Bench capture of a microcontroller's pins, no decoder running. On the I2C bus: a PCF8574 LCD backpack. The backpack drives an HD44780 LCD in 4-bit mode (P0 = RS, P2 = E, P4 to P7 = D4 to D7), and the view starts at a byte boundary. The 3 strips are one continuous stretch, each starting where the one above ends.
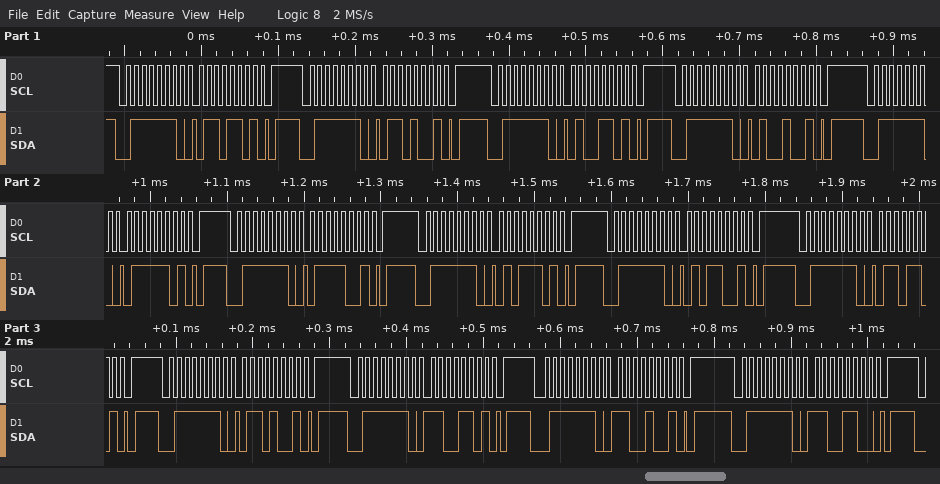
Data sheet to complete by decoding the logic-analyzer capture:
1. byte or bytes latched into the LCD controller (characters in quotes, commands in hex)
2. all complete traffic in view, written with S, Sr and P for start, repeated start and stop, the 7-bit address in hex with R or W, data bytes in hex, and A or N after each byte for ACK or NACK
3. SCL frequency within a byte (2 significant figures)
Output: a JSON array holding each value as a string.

["'d' 'u' 'l'", "S 3FW A 6D A P S 3FW A 69 A P S 3FW A 4D A P S 3FW A 49 A P S 3FW A 7D A P S 3FW A 79 A P S 3FW A 5D A P S 3FW A 59 A P S 3FW A 6D A P S 3FW A 69 A P S 3FW A CD A P S 3FW A C9 A P S 3FW A CC A P", "100 kHz"]
